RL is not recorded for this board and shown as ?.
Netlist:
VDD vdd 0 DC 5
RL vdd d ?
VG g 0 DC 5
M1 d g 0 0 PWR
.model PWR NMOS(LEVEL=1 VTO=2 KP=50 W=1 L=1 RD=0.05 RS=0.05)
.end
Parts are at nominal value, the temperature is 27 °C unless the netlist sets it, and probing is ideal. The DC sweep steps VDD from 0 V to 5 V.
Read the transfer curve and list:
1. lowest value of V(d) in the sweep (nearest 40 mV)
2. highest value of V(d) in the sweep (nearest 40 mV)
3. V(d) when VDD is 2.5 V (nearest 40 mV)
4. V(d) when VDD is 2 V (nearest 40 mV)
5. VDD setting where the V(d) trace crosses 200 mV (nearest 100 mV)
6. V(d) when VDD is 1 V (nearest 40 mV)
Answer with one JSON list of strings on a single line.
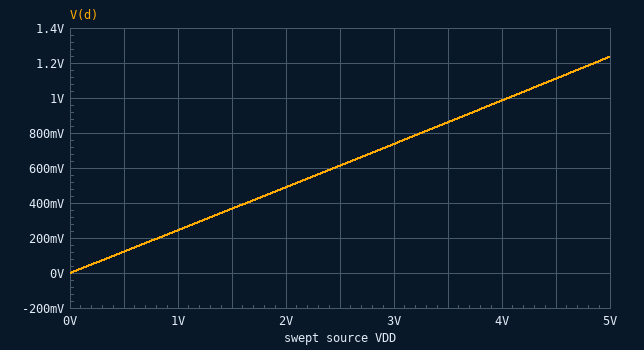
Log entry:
["0 V", "1.24 V", "600 mV", "480 mV", "800 mV", "240 mV"]
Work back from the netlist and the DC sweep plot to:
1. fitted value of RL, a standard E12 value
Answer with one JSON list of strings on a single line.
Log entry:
["0.33 Ω"]
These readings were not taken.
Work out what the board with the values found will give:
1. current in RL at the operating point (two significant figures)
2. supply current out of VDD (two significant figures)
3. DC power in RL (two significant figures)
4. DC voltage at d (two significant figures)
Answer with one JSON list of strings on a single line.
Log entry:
["11 A", "11 A", "43 W", "1.2 V"]
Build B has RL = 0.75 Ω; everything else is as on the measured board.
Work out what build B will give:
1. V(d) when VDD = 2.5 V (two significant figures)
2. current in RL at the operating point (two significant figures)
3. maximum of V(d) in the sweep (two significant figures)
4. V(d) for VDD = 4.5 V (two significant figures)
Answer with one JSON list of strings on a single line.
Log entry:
["310 mV", "5.8 A", "630 mV", "560 mV"]
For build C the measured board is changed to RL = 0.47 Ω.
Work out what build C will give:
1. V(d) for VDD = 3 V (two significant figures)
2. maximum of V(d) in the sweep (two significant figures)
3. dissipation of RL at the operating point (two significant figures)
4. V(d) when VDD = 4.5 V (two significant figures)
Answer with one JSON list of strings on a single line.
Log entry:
["560 mV", "930 mV", "35 W", "840 mV"]
